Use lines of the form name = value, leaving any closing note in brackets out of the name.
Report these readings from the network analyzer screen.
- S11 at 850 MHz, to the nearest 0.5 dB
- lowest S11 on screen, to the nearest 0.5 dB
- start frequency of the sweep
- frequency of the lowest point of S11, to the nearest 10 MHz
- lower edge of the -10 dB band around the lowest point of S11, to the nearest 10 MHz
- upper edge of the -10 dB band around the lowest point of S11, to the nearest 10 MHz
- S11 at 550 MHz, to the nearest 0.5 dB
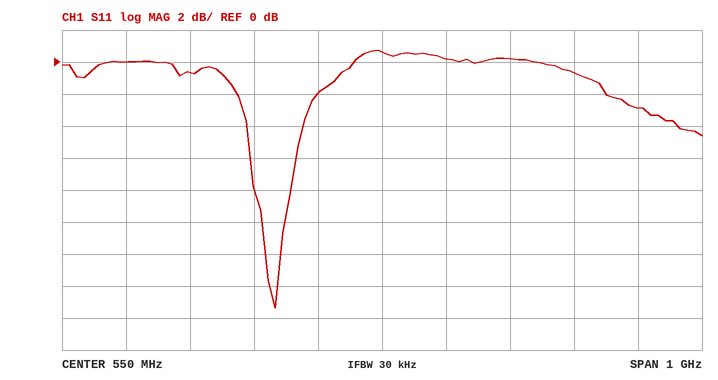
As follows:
S11 at 850 MHz, to the nearest 0.5 dB = -0.5 dB
lowest S11 on screen, to the nearest 0.5 dB = -15.5 dB
start frequency of the sweep = 50 MHz
frequency of the lowest point of S11, to the nearest 10 MHz = 380 MHz
lower edge of the -10 dB band around the lowest point of S11, to the nearest 10 MHz = 360 MHz
upper edge of the -10 dB band around the lowest point of S11, to the nearest 10 MHz = 400 MHz
S11 at 550 MHz, to the nearest 0.5 dB = 0.5 dB
